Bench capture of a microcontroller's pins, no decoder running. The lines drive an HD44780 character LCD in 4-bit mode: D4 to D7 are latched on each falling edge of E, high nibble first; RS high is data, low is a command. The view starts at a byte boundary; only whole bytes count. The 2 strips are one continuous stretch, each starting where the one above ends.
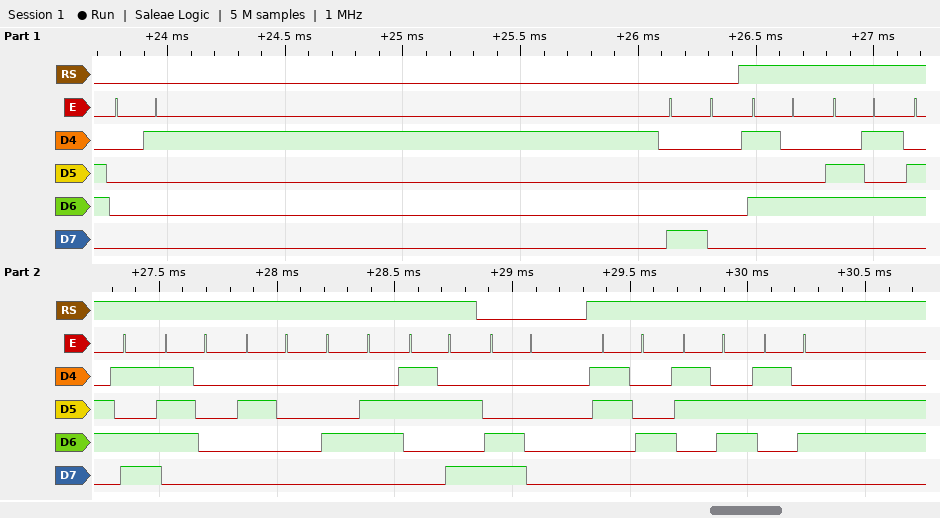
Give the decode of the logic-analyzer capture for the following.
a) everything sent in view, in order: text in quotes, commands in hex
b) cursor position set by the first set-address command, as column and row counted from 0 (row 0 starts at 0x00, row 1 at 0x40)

0x01 0x80 "Temp F:" 0xC0 "466"
column 0, row 0
